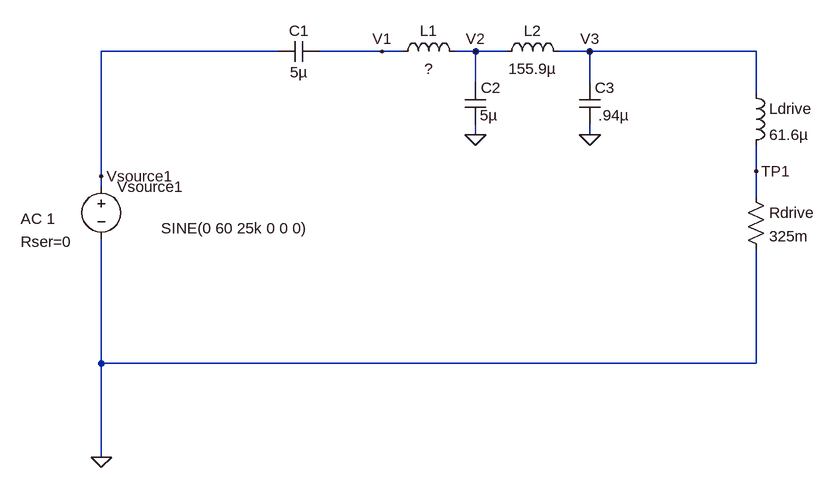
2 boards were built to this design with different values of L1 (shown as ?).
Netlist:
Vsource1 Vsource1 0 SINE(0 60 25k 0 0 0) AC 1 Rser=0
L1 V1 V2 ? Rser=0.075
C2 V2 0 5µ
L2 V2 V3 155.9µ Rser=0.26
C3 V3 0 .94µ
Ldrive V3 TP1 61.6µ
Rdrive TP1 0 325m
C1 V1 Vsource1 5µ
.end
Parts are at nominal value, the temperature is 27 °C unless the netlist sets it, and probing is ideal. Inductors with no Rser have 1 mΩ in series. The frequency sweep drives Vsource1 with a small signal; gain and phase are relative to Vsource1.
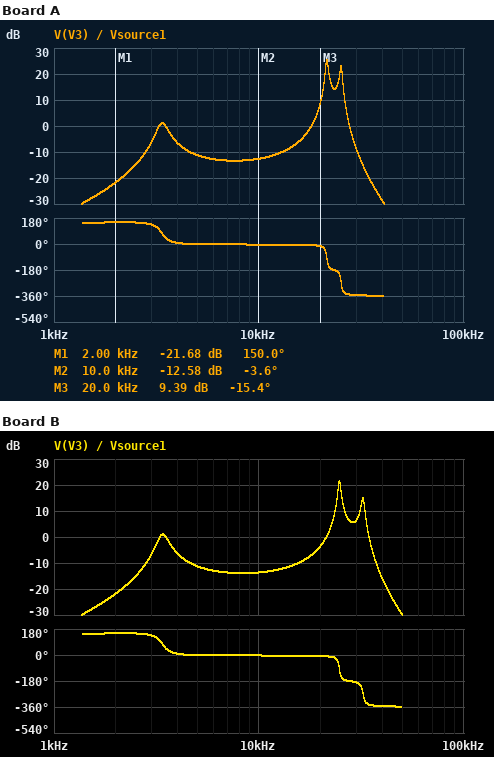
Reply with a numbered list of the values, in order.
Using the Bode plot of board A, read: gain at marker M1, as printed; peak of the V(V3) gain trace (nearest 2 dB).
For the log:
1. -21.68 dB
2. 26 dB
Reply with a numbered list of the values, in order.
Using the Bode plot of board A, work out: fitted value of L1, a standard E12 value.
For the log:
1. 22 µH
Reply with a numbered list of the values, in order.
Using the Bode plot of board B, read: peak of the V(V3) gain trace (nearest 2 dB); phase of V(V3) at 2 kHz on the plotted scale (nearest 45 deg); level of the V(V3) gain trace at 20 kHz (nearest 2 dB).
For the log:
1. 22 dB
2. 135 deg
3. -4 dB
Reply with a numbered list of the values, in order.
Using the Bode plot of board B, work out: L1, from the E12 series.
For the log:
1. 10 µH
